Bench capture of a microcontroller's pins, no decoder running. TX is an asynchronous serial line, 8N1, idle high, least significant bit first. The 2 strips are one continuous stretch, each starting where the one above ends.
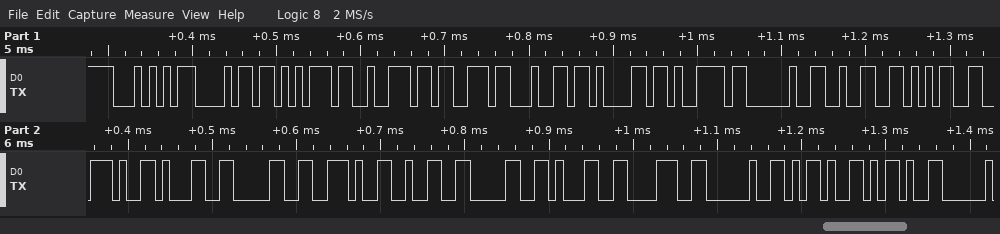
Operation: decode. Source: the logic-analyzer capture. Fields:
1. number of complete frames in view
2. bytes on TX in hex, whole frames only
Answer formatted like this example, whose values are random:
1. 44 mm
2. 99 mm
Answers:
1. 22
2. 0x54 0x68 0x75 0x72 0x73 0x64 0x61 0x79 0x20 0x32 0x35 0x2E 0x31 0x30 0x2E 0x32 0x30 0x31 0x38 0x20 0x2D 0x2D
